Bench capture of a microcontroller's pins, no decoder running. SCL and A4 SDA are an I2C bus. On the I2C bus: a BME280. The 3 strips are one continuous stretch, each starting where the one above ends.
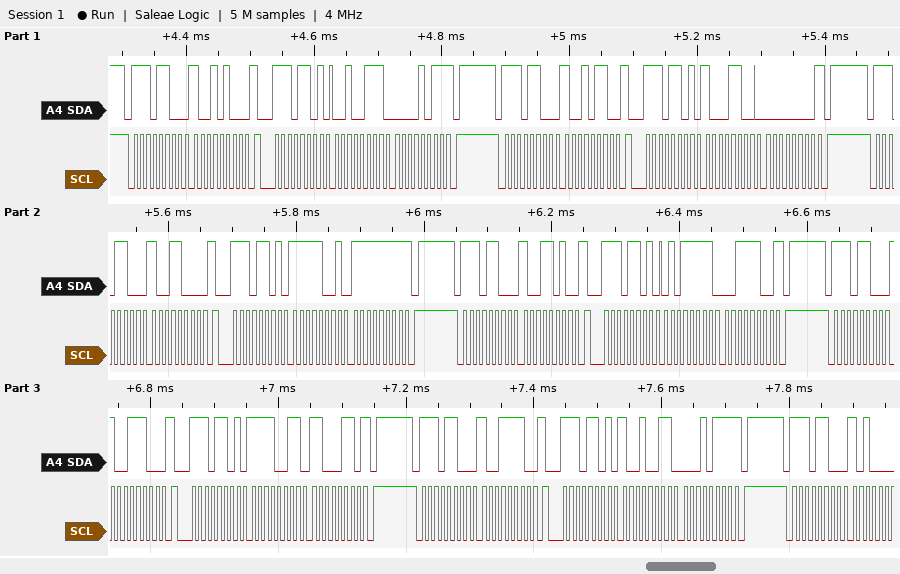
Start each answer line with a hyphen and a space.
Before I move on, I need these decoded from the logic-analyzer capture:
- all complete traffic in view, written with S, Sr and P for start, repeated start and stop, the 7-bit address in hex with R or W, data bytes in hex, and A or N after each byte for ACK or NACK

- S 76W A 94 A Sr 76R A 27 A 0B N P S 76W A 96 A Sr 76R A 8C A 00 N P S 76W A 98 A Sr 76R A F9 A FF N P S 76W A 9A A Sr 76R A 5F A 3C N P S 76W A 9C A Sr 76R A F3 A C6 N P S 76W A 9E A Sr 76R A 93 A 17 N P S 76W A
